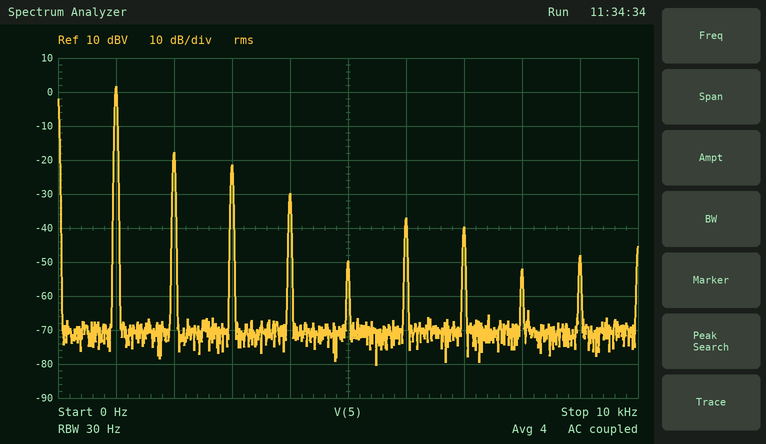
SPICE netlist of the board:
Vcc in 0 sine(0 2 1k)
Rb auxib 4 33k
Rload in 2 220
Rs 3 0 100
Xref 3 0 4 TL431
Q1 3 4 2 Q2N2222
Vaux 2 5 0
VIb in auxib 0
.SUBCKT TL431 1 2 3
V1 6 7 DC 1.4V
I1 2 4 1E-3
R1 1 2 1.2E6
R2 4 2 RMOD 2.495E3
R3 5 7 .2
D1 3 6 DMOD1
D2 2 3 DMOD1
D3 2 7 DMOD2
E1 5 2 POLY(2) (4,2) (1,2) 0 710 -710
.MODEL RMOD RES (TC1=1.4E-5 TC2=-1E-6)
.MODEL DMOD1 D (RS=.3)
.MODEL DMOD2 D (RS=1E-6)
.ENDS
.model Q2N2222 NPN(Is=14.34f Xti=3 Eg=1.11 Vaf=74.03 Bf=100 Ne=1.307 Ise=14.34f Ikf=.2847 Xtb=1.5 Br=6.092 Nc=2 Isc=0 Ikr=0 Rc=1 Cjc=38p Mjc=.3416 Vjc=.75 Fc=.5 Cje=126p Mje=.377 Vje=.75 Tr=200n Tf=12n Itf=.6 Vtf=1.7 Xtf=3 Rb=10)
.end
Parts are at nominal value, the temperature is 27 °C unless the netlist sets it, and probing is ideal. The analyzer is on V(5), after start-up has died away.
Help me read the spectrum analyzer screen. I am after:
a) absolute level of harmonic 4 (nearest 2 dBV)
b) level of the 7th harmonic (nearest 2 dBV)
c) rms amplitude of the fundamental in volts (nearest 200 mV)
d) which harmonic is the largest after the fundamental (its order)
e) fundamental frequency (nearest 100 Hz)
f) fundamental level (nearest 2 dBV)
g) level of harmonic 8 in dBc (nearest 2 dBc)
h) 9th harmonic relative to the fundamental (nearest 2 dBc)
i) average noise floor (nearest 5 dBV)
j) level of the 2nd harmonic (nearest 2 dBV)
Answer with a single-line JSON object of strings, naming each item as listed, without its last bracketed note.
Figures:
{"absolute level of harmonic 4": "-30 dBV", "level of the 7th harmonic": "-40 dBV", "rms amplitude of the fundamental in volts": "1.2 V", "which harmonic is the largest after the fundamental": "2", "fundamental frequency": "1.0 kHz", "fundamental level": "2 dBV", "level of harmonic 8 in dBc": "-54 dBc", "9th harmonic relative to the fundamental": "-50 dBc", "average noise floor": "-70 dBV", "level of the 2nd harmonic": "-18 dBV"}
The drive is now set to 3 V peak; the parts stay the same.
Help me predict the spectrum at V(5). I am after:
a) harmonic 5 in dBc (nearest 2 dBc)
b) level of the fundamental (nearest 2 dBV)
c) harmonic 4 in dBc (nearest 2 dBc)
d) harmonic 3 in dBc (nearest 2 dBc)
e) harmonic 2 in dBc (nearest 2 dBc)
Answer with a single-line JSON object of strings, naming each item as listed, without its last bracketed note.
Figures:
{"harmonic 5 in dBc": "-32 dBc", "level of the fundamental": "4 dBV", "harmonic 4 in dBc": "-54 dBc", "harmonic 3 in dBc": "-22 dBc", "harmonic 2 in dBc": "-14 dBc"}
